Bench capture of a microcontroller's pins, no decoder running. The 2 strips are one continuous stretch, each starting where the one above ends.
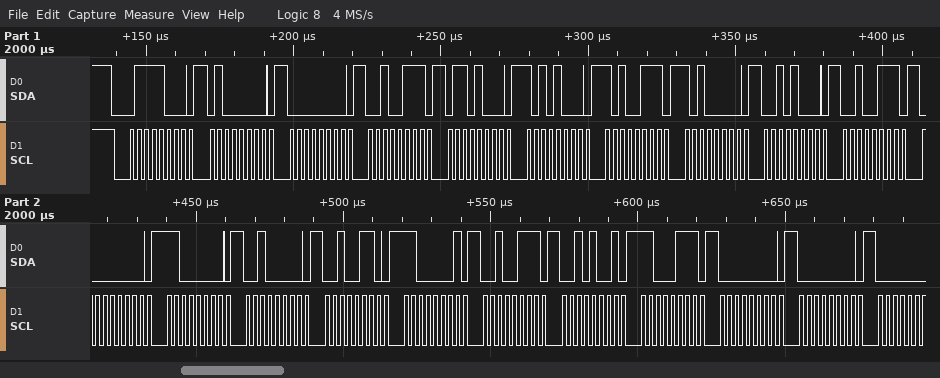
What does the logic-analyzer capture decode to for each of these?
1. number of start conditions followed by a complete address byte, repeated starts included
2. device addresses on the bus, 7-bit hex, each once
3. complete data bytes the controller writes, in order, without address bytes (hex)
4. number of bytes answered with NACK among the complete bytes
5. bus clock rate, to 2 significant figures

1
0x3C
40 00 27 68 A8 A7 A0 28 27 00 C0 20 26 C1 27 29 C7 00 00
0
400 kHz
